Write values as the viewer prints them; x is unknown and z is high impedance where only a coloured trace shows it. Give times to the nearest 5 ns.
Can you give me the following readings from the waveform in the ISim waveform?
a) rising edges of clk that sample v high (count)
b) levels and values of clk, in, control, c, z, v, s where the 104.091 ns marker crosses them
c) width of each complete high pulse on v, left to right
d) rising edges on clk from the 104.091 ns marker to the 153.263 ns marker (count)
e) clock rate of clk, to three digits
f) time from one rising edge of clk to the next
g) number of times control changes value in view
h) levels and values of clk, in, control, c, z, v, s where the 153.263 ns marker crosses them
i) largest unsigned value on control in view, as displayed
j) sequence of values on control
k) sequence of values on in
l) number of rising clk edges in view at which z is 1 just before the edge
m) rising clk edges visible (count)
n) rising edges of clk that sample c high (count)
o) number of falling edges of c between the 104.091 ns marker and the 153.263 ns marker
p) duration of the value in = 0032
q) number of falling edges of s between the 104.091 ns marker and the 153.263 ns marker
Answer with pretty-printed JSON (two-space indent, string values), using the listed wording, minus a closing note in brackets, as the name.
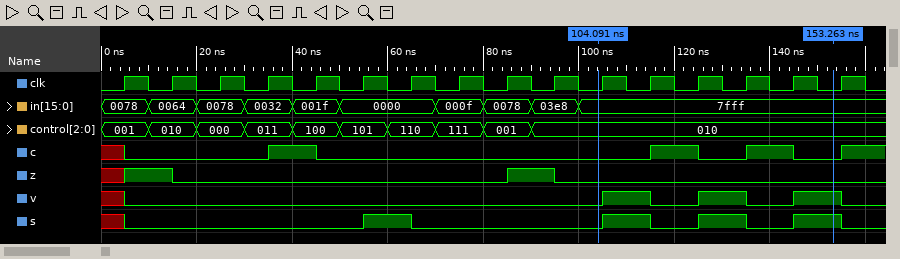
{
  "rising edges of clk that sample v high": "3",
  "levels and values of clk, in, control, c, z, v, s where the 104.091 ns marker crosses them": "clk=0, in=7fff, control=010, c=0, z=0, v=0, s=0",
  "width of each complete high pulse on v, left to right": "10 ns, 10 ns, 10 ns",
  "rising edges on clk from the 104.091 ns marker to the 153.263 ns marker": "5",
  "clock rate of clk, to three digits": "100 MHz",
  "time from one rising edge of clk to the next": "10 ns",
  "number of times control changes value in view": "9",
  "levels and values of clk, in, control, c, z, v, s where the 153.263 ns marker crosses them": "clk=0, in=7fff, control=010, c=0, z=0, v=1, s=1",
  "largest unsigned value on control in view, as displayed": "111",
  "sequence of values on control": "001, 010, 000, 011, 100, 101, 110, 111, 001, 010",
  "sequence of values on in": "0078, 0064, 0078, 0032, 001f, 0000, 000f, 0078, 03e8, 7fff",
  "number of rising clk edges in view at which z is 1 just before the edge": "2",
  "rising clk edges visible": "16",
  "rising edges of clk that sample c high": "3",
  "number of falling edges of c between the 104.091 ns marker and the 153.263 ns marker": "2",
  "duration of the value in = 0032": "10 ns",
  "number of falling edges of s between the 104.091 ns marker and the 153.263 ns marker": "2"
}
